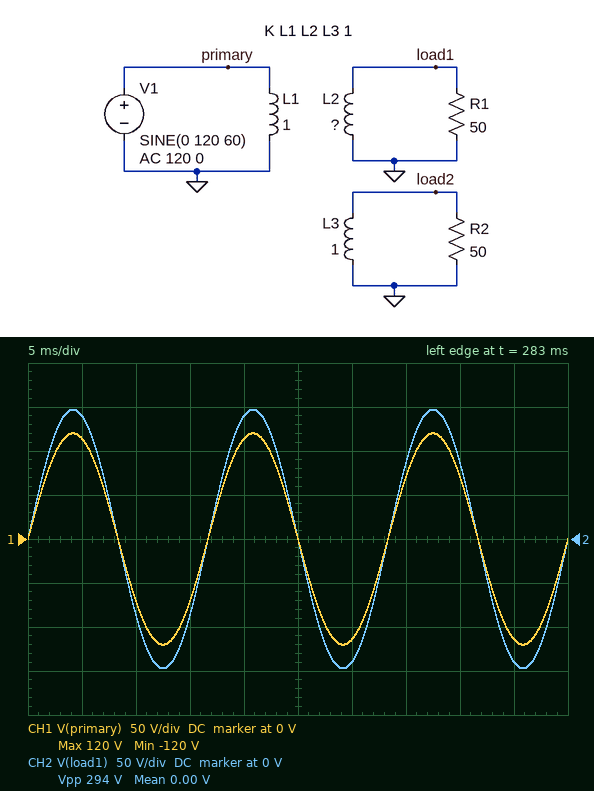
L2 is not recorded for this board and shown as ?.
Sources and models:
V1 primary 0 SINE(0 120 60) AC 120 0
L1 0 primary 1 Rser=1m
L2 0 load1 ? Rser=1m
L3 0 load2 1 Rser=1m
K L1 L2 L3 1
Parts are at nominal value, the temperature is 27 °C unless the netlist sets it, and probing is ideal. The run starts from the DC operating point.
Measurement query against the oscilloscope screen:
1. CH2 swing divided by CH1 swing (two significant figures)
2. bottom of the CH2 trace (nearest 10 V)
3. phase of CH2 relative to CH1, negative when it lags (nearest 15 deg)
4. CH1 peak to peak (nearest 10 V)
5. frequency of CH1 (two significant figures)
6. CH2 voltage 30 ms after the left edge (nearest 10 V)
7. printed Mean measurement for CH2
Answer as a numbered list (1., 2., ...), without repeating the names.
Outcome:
1. 1.2
2. -150 V
3. 0 deg
4. 240 V
5. 60 Hz
6. -140 V
7. 0.00 V
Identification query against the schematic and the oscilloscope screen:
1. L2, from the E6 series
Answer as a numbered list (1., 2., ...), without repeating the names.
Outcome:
1. 1.5 H
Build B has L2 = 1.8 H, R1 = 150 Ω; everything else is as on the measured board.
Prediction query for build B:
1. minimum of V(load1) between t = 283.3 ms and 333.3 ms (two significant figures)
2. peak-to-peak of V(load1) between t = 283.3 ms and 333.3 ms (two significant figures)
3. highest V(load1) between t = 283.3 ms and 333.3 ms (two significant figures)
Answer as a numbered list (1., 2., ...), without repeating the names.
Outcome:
1. -160 V
2. 320 V
3. 160 V
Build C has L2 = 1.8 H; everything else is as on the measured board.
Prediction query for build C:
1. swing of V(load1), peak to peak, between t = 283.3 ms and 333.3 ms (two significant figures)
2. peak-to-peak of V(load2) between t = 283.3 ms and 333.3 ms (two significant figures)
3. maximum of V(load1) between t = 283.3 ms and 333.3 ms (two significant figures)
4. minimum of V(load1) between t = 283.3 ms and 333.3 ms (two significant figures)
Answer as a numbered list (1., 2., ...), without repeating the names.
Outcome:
1. 320 V
2. 240 V
3. 160 V
4. -160 V
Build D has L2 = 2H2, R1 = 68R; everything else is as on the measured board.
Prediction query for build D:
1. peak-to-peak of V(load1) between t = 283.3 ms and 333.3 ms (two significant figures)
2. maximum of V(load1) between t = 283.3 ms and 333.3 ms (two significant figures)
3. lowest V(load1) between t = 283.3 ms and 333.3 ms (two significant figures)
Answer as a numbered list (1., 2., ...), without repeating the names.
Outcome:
1. 360 V
2. 180 V
3. -180 V
